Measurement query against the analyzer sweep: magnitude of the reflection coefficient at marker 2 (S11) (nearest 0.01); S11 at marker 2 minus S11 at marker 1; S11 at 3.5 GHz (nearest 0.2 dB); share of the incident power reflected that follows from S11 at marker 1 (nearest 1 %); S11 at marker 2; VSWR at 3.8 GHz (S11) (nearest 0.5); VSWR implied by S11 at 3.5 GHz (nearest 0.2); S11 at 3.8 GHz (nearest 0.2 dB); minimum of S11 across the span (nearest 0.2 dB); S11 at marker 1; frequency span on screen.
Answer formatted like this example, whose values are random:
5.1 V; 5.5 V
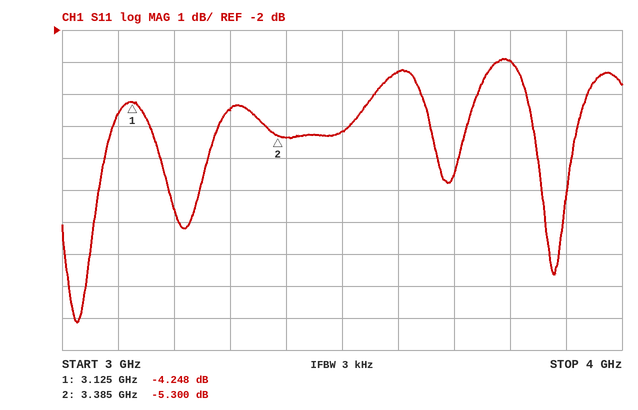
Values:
0.54; -1.052 dB; -5.2 dB; 38 %; -5.300 dB; 6.0; 3.4; -3.0 dB; -11.2 dB; -4.248 dB; 1 GHz
